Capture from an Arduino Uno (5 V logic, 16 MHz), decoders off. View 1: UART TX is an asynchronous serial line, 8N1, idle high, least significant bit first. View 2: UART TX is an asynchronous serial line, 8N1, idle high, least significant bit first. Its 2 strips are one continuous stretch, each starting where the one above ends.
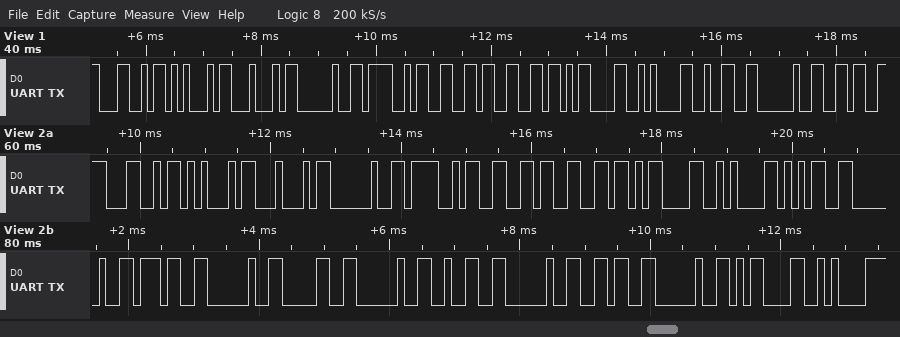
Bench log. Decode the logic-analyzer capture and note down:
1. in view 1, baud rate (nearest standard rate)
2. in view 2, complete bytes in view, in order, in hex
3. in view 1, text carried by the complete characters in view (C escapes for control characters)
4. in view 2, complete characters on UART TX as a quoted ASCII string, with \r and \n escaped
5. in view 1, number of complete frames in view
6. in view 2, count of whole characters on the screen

9600 baud
4C 45 44 20 4F 66 66 0D 0A 35 20 37 20 30 20 32 20 36 20 0D 0A
"LED Off\r\n2 6"
"LED Off\r\n5 7 0 2 6 \r\n"
12
21
